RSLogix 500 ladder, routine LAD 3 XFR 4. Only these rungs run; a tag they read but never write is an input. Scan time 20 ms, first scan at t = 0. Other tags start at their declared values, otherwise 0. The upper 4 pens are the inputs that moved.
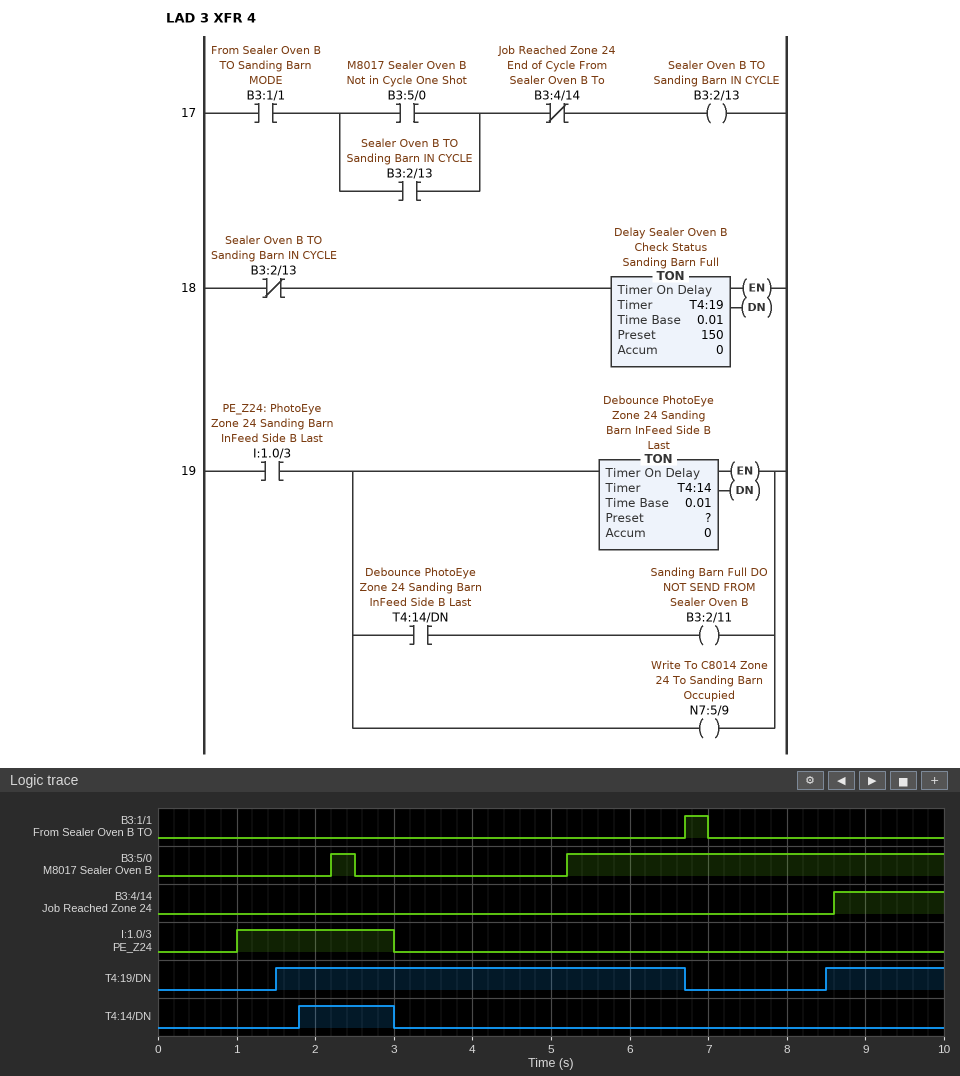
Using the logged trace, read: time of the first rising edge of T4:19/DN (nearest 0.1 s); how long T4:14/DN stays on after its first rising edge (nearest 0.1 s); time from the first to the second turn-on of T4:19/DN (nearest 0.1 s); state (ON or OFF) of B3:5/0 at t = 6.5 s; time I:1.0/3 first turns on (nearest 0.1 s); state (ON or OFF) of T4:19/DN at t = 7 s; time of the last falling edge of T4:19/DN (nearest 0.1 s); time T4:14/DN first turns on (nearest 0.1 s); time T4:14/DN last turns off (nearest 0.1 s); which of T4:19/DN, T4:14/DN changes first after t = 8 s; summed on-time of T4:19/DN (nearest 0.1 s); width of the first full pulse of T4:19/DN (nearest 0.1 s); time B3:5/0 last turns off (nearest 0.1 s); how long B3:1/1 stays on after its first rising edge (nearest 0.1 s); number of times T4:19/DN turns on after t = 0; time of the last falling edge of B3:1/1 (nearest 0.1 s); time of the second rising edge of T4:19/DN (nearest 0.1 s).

1.5 s
1.2 s
7.0 s
ON
1.0 s
OFF
6.7 s
1.8 s
3.0 s
T4:19/DN
6.7 s
5.2 s
2.5 s
0.3 s
2
7.0 s
8.5 s
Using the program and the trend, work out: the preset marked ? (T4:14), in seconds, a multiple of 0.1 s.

0.8 s
